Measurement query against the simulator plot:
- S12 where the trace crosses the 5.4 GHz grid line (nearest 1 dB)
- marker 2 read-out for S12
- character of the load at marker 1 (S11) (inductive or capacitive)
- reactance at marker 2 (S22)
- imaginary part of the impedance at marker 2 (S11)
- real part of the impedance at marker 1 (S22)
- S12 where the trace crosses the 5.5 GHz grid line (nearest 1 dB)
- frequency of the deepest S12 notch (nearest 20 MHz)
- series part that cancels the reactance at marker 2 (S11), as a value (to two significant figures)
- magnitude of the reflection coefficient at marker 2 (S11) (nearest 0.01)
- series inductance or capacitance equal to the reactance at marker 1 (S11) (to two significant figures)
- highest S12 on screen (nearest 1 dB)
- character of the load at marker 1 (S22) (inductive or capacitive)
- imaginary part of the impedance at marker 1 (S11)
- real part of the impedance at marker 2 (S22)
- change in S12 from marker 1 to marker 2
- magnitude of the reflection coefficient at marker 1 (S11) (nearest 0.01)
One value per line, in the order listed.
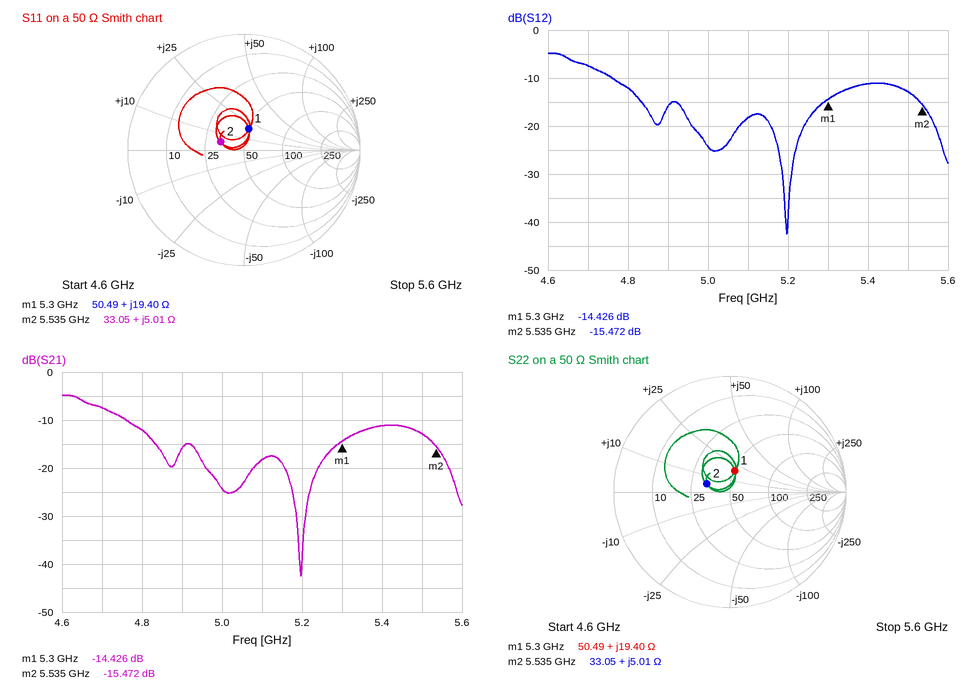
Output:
-11 dB
-15.472 dB
inductive
+5.01 Ω
+5.01 Ω
50.49 Ω
-13 dB
5.20 GHz
5.7 pF
0.21
580 pH
-5 dB
inductive
+19.40 Ω
33.05 Ω
-1.046 dB
0.19
